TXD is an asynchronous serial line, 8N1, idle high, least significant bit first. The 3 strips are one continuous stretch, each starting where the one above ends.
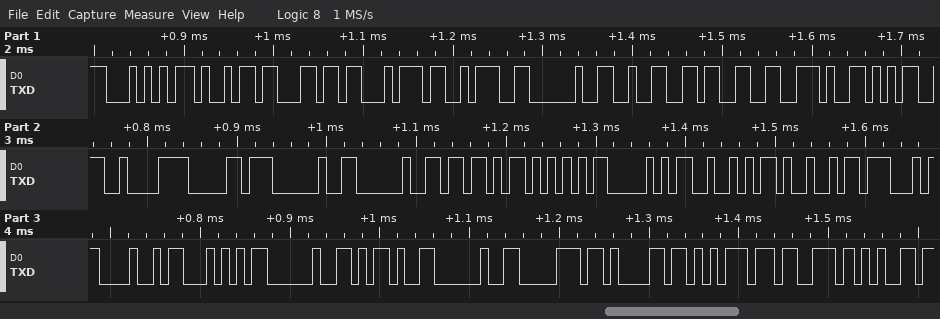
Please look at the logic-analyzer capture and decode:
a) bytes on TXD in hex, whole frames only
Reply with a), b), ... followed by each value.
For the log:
a) 54 69 6C 74 3A 20 32 33 2E 35 C2 B0 20 20 5B 55 50 52 49 47 48 54 20 2D 20 70 61 75 73 65
